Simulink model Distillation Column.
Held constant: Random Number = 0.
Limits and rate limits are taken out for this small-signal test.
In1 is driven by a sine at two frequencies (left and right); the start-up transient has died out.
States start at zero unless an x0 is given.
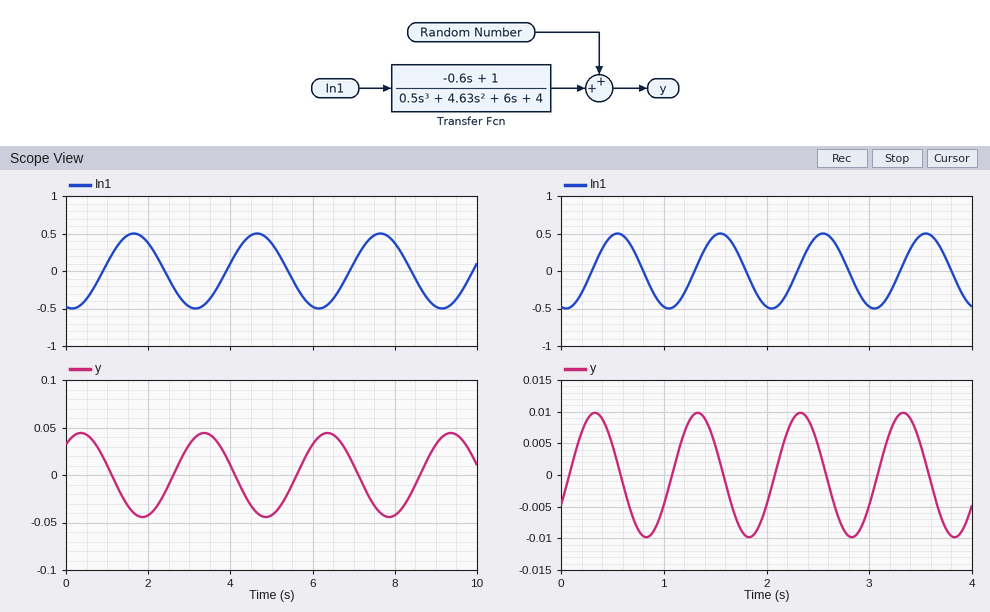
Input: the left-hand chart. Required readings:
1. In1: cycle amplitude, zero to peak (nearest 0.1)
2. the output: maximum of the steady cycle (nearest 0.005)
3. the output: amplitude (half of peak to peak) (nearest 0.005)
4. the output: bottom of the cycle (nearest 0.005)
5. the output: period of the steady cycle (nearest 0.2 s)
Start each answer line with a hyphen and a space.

- 0.5
- 0.045
- 0.045
- -0.045
- 3.0 s
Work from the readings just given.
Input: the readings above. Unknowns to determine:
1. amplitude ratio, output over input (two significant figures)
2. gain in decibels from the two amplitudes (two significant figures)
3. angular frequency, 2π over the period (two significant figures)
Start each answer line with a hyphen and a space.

- 0.090
- -21 dB
- 2.1 rad/s
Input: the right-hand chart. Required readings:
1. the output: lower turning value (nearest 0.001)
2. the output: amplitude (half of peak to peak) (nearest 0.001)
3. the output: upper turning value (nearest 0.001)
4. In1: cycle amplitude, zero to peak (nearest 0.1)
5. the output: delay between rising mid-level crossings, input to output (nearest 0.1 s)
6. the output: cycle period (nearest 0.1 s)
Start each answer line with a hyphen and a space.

- -0.010
- 0.010
- 0.010
- 0.5
- 0.8 s
- 1.0 s
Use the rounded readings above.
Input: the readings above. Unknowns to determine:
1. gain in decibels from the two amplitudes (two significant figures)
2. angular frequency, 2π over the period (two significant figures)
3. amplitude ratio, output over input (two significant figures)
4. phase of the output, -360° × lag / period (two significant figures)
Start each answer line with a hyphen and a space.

- -34 dB
- 6.3 rad/s
- 0.020
- -290°
